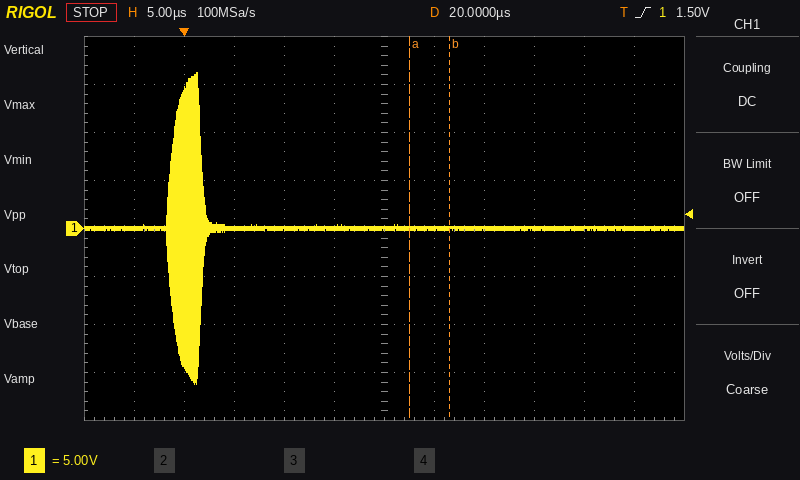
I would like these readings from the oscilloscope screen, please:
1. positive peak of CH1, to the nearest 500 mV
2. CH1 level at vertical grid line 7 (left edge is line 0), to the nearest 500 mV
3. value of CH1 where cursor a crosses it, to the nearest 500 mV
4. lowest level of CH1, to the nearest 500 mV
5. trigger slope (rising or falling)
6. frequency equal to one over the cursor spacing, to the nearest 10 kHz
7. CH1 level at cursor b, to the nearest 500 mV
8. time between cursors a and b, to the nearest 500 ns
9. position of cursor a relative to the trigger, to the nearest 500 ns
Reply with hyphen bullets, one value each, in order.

- 16.0 V
- 0.0 V
- 0.0 V
- -16.0 V
- rising
- 250 kHz
- 0.0 V
- 4.0 µs
- +22.5 µs
